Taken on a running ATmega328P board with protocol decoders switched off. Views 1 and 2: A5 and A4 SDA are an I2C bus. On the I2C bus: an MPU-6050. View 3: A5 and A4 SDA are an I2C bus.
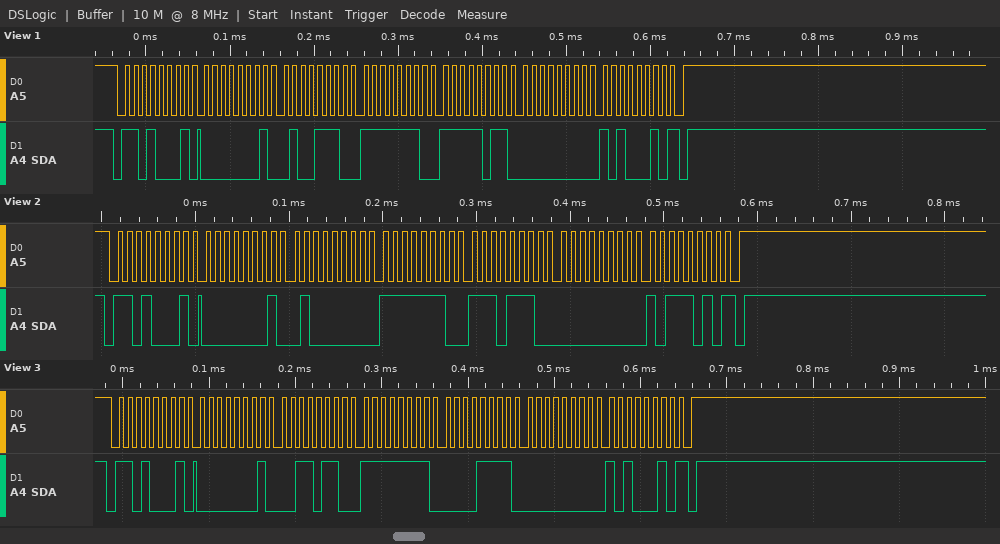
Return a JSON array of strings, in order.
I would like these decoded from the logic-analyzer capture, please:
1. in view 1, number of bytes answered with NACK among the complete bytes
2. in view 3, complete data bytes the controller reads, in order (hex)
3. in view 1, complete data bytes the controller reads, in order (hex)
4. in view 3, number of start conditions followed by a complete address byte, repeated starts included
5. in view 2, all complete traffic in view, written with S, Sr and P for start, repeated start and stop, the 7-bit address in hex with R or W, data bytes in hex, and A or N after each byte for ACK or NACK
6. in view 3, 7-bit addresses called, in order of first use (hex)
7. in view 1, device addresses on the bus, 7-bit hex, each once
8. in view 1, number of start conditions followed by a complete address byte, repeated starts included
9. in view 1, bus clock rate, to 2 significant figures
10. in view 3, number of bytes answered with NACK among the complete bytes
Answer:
["1", "01 36 FF 0F 00 A2", "01 4E FE FB 00 A2", "1", "S 68R A 01 A 40 A FE A EE A 00 A BA N P", "0x68", "0x68", "1", "100 kHz", "1"]
